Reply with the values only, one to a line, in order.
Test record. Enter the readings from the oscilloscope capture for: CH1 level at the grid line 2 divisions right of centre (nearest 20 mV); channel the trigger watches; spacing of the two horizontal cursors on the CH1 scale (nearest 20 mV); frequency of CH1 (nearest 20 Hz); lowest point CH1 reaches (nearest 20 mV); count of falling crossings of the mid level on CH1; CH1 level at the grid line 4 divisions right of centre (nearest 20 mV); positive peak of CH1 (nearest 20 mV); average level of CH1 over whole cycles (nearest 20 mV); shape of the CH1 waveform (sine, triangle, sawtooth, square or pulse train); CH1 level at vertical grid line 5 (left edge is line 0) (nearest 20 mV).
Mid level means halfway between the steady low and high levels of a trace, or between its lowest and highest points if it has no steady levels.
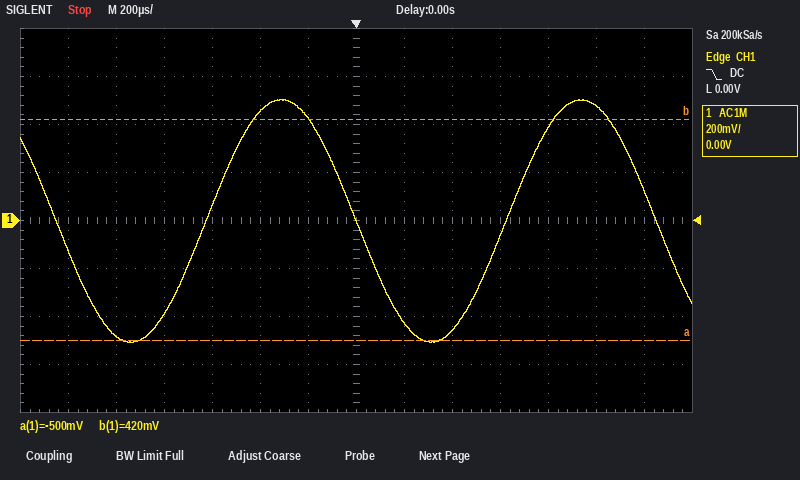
-460 mV
CH1
920 mV
800 Hz
-500 mV
3
380 mV
500 mV
0 mV
sine
460 mV
